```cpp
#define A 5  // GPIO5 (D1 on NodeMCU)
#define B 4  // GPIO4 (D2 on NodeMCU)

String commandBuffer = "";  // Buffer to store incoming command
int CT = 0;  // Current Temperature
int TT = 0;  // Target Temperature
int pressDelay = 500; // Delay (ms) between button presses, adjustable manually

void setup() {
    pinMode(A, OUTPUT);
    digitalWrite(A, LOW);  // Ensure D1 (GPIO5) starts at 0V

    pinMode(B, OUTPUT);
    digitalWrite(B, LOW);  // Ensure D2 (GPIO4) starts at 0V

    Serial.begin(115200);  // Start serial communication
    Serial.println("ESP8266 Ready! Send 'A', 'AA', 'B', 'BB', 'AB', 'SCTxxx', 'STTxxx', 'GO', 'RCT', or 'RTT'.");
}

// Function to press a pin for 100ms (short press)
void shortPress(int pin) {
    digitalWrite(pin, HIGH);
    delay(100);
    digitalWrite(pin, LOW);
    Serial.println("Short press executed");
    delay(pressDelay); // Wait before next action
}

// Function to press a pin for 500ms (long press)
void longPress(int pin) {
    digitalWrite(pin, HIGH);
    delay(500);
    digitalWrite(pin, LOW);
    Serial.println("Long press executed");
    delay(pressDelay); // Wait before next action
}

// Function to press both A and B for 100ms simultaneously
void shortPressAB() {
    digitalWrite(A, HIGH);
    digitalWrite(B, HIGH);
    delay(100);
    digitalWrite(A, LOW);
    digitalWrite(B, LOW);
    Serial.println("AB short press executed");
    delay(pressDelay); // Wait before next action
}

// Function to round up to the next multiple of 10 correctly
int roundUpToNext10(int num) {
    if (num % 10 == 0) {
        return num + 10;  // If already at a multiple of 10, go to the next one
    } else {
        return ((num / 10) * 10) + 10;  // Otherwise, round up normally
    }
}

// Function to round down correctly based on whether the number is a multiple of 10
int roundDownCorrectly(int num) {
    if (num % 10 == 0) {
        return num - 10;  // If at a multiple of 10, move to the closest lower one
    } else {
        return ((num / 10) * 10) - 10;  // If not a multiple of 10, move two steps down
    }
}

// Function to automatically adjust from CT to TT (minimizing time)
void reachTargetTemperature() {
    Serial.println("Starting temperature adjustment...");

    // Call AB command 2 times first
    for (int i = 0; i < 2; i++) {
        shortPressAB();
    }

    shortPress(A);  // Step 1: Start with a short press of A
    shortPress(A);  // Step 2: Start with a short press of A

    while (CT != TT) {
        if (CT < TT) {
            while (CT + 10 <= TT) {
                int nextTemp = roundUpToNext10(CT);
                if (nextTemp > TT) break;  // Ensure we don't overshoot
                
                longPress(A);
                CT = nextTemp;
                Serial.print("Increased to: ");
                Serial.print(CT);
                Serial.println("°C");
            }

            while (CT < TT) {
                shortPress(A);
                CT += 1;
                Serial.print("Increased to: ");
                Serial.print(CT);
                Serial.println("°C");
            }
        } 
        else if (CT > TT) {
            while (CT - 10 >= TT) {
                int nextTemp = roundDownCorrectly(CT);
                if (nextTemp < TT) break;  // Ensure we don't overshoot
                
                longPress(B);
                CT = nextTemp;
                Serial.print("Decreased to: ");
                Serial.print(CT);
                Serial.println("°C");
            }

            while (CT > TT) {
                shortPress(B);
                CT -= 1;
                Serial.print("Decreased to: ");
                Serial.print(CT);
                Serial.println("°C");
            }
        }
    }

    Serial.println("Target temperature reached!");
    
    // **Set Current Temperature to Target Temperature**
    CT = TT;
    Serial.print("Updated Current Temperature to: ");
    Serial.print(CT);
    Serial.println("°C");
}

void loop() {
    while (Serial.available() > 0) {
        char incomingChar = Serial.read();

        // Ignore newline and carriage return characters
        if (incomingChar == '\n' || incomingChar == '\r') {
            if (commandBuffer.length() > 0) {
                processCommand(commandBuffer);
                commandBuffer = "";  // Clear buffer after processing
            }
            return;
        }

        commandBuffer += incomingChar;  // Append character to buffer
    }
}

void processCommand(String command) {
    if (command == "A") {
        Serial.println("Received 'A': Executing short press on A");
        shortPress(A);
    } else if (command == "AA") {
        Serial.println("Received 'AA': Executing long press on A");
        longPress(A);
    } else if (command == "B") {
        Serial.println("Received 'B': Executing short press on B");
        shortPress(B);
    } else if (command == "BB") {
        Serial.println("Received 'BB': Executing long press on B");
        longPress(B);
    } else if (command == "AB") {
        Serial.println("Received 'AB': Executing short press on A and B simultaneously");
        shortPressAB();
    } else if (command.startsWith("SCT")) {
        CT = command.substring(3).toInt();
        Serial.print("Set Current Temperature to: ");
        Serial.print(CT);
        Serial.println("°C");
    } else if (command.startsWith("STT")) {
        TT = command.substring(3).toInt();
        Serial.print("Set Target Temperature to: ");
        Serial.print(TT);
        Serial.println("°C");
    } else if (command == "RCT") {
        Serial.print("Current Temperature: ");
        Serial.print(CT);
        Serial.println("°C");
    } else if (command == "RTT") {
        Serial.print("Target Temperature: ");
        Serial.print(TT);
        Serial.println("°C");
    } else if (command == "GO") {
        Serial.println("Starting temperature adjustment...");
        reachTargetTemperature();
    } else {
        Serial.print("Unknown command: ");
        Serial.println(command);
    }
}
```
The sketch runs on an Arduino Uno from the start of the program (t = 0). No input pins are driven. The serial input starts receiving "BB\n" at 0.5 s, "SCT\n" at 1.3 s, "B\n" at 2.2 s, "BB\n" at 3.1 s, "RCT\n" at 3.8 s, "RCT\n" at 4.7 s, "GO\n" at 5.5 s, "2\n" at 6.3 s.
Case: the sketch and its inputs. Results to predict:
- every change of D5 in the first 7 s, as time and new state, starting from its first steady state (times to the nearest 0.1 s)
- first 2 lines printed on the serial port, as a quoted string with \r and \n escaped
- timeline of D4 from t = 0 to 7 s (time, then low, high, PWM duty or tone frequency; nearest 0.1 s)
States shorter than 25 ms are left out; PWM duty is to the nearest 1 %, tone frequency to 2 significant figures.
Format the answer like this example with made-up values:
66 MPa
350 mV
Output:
0 s low; 5.5 s high; 5.6 s low; 6.1 s high; 6.2 s low; 6.7 s high; 6.8 s low
"ESP8266 Ready! Send 'A', 'AA', 'B', 'BB', 'AB', 'SCTxxx', 'STTxxx', 'GO', 'RCT', or 'RTT'.\r\nReceived 'BB': Executing long press on B\r\n"
0 s low; 0.5 s high; 1 s low; 2.2 s high; 2.3 s low; 3.1 s high; 3.6 s low; 5.5 s high; 5.6 s low; 6.1 s high; 6.2 s low
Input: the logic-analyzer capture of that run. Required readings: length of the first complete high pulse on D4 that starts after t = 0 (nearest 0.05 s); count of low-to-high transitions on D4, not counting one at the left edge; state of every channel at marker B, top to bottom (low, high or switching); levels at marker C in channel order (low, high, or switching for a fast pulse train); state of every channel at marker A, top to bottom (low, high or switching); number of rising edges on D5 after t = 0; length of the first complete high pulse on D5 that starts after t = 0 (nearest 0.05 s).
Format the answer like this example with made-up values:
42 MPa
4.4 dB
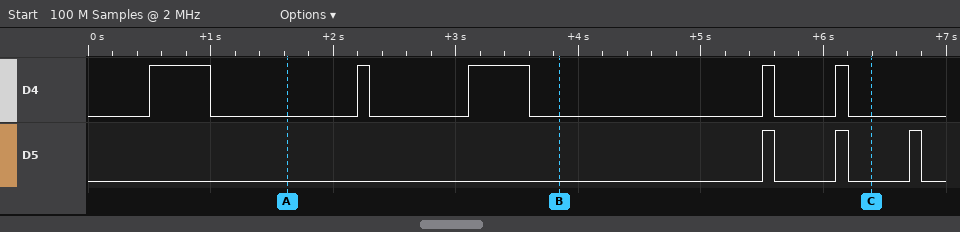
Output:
0.50 s
5
D4 low, D5 low
D4 low, D5 low
D4 low, D5 low
3
0.10 s
